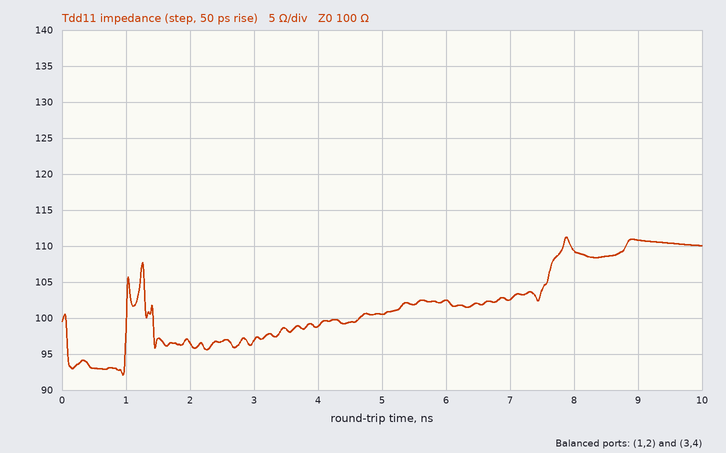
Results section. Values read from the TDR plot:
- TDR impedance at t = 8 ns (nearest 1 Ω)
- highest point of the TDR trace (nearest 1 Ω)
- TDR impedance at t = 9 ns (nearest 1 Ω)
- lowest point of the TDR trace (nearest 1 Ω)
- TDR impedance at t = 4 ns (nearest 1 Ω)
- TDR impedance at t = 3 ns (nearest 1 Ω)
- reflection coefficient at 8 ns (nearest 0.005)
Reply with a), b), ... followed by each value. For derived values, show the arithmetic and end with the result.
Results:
a) 109 Ω
b) 111 Ω
c) 111 Ω
d) 92 Ω
e) 99 Ω
f) 97 Ω
g) (109 − 100)/(109 + 100) ≈ +0.0431, so +0.045 to the nearest 0.005
